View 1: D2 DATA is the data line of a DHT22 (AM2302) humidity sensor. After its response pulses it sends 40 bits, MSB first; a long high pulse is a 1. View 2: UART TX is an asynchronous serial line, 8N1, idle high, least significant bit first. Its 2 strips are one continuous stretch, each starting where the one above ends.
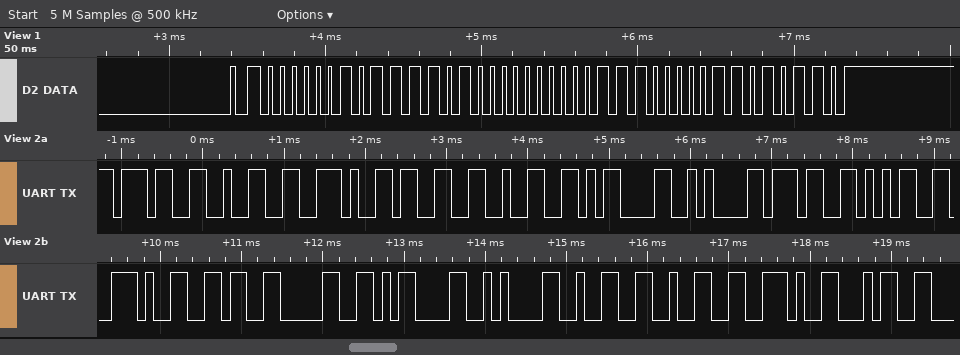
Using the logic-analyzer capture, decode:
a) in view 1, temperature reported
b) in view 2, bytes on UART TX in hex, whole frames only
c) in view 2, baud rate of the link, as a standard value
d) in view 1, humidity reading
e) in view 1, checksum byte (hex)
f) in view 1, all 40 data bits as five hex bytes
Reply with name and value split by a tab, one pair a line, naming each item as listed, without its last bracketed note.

in view 1, temperature reported	22.4 °C
in view 2, bytes on UART TX in hex, whole frames only	37 32 2E 33 32 0D 0A 37 35 2E 36 30 0D 0A 32 32 2E 34
in view 2, baud rate of the link, as a standard value	9600 baud
in view 1, humidity reading	75.6 %
in view 1, checksum byte	0xD6
in view 1, all 40 data bits as five hex bytes	02 F4 00 E0 D6
